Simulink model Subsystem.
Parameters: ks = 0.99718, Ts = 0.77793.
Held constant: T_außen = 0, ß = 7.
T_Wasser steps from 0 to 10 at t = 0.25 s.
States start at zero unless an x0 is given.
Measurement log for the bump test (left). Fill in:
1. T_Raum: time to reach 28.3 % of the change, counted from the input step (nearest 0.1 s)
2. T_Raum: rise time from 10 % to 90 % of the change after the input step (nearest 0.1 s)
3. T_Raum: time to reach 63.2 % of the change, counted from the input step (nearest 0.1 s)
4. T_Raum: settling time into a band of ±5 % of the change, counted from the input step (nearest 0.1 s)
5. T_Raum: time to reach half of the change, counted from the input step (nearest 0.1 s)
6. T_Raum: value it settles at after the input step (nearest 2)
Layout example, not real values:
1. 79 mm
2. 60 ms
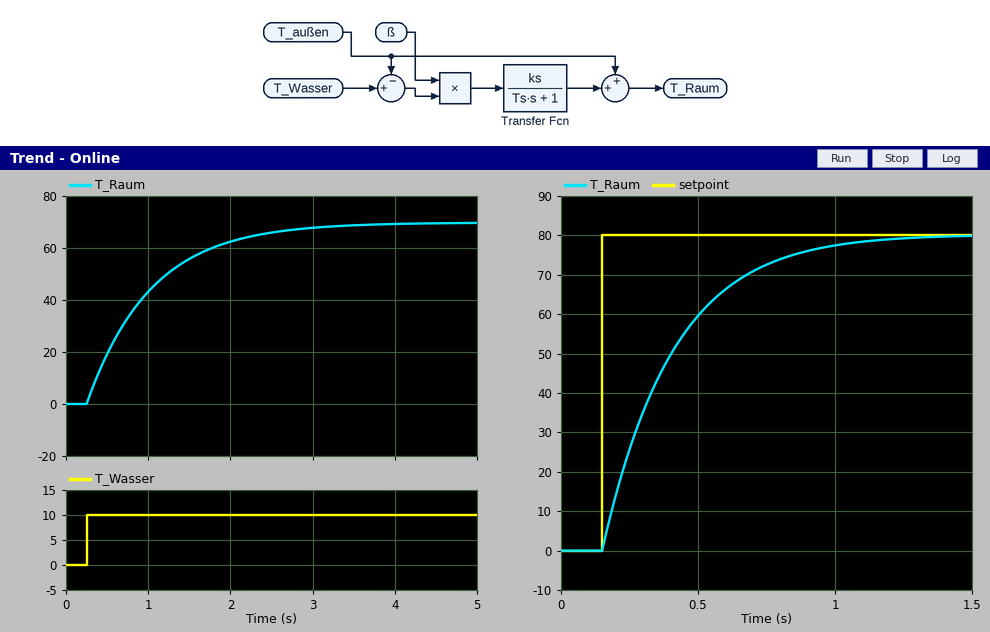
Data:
1. 0.3 s
2. 1.7 s
3. 0.8 s
4. 2.3 s
5. 0.5 s
6. 70
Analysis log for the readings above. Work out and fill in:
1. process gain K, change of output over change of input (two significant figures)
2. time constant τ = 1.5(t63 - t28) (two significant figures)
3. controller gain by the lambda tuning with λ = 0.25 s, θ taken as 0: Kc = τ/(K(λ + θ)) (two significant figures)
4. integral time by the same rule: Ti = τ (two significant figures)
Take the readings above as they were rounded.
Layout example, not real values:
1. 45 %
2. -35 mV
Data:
1. 7.0
2. 0.75 s
3. 0.43
4. 0.75 s
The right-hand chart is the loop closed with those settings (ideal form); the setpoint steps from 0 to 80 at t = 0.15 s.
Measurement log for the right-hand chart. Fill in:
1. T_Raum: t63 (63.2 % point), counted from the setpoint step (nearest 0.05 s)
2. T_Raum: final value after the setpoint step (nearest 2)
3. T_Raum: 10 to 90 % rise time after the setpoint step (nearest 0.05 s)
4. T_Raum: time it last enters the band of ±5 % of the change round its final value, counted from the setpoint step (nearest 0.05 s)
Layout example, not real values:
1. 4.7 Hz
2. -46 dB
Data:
1. 0.25 s
2. 80
3. 0.55 s
4. 0.75 s
